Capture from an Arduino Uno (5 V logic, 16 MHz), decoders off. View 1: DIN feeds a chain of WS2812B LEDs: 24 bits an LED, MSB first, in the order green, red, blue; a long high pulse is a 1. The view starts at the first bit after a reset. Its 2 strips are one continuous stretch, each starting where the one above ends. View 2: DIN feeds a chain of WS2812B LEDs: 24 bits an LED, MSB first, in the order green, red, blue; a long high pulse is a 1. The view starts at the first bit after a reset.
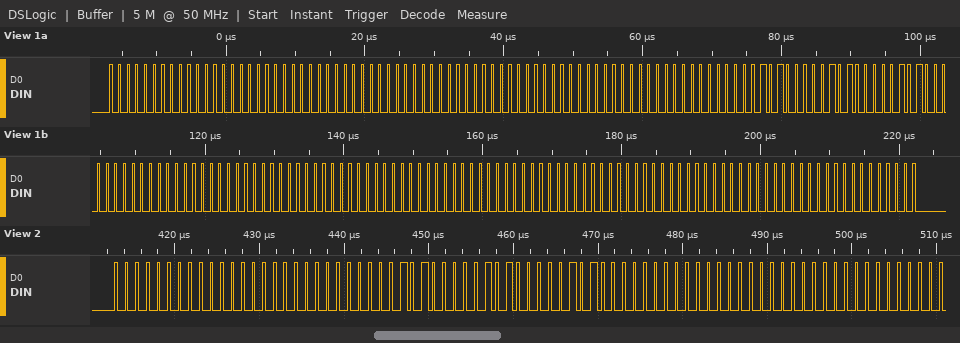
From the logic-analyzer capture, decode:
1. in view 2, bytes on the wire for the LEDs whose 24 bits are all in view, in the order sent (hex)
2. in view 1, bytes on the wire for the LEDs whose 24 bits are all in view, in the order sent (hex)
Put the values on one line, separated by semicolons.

00 00 00 14 14 14 00 00 00; 00 00 00 00 00 00 00 00 00 14 14 14 00 00 00 00 00 00 00 00 00 00 00 00
